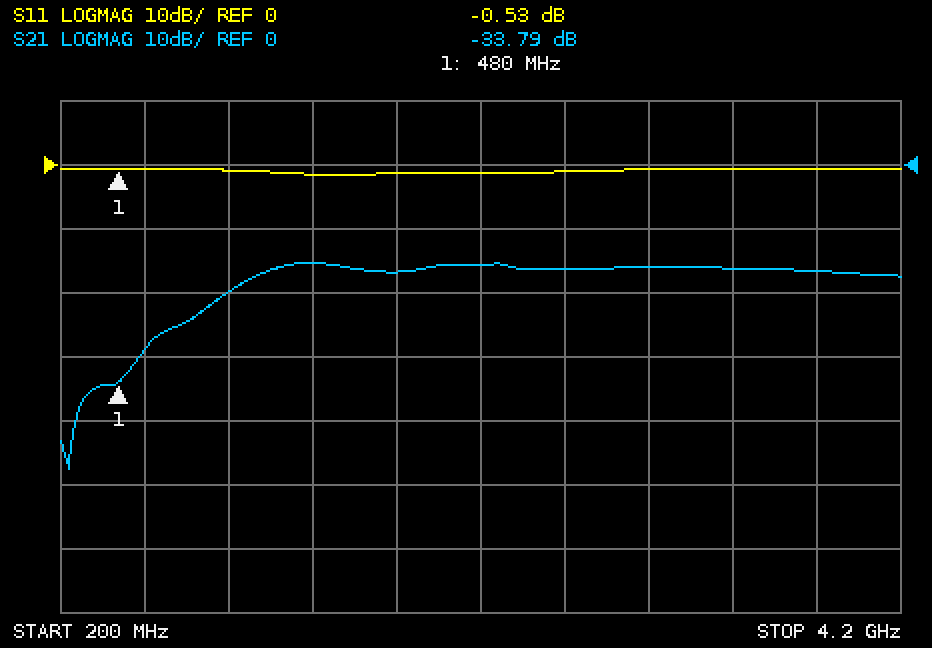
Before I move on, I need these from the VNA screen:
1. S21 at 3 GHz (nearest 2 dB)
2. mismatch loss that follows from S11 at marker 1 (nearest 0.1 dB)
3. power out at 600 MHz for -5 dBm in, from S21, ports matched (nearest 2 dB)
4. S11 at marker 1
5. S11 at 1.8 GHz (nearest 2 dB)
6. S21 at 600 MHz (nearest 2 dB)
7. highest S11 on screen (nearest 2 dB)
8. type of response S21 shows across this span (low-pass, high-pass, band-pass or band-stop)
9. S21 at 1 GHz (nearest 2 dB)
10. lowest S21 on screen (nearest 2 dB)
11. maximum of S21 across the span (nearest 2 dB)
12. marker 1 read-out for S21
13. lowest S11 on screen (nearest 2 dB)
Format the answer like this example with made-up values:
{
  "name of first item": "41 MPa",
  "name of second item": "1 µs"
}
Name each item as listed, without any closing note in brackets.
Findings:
{
  "S21 at 3 GHz": "-16 dB",
  "mismatch loss that follows from S11 at marker 1": "9.4 dB",
  "power out at 600 MHz for -5 dBm in, from S21, ports matched": "-34 dBm",
  "S11 at marker 1": "-0.53 dB",
  "S11 at 1.8 GHz": "-2 dB",
  "S21 at 600 MHz": "-28 dB",
  "highest S11 on screen": "0 dB",
  "type of response S21 shows across this span": "high-pass",
  "S21 at 1 GHz": "-20 dB",
  "lowest S21 on screen": "-48 dB",
  "maximum of S21 across the span": "-16 dB",
  "marker 1 read-out for S21": "-33.79 dB",
  "lowest S11 on screen": "-2 dB"
}
